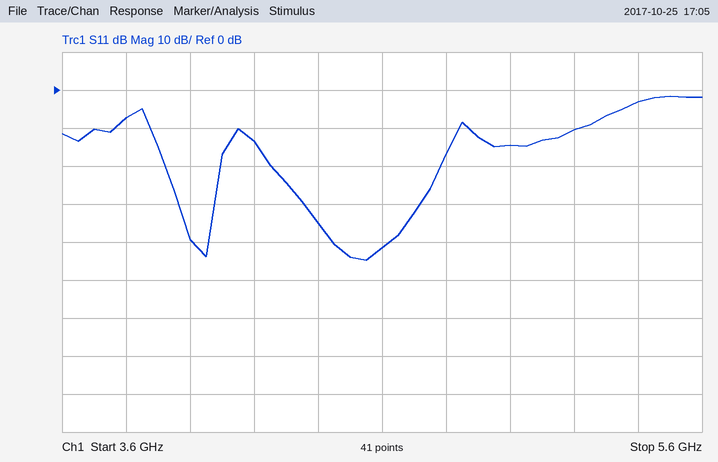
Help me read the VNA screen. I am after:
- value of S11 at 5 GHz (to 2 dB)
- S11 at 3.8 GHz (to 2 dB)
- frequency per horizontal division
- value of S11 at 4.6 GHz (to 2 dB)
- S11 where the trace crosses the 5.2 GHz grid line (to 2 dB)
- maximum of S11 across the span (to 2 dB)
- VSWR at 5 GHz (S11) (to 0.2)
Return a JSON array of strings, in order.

["-14 dB", "-8 dB", "200 MHz", "-42 dB", "-10 dB", "-2 dB", "1.4"]
